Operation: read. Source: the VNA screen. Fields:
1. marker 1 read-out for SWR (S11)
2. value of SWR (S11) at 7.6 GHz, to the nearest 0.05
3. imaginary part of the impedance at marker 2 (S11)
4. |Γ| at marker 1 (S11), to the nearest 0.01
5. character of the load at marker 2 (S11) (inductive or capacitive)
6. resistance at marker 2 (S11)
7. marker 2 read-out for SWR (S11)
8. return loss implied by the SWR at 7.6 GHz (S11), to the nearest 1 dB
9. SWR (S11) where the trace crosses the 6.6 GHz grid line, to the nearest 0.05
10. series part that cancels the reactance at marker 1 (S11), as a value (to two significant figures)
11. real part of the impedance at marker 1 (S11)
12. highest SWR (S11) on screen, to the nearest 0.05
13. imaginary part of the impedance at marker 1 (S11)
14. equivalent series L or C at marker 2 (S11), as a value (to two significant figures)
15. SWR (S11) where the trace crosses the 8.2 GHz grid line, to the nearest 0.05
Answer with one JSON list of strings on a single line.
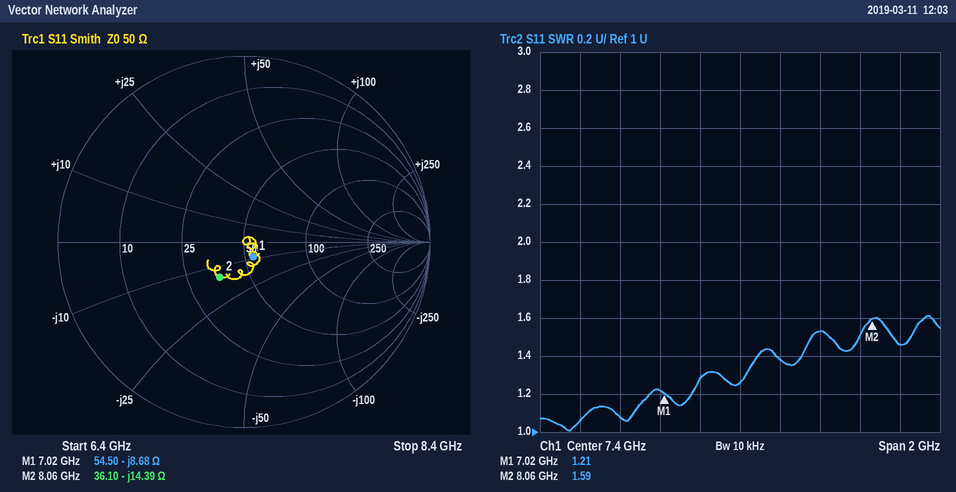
["1.21", "1.40", "-14.39 Ω", "0.09", "capacitive", "36.10 Ω", "1.59", "16 dB", "1.05", "200 pH", "54.50 Ω", "1.60", "-8.68 Ω", "1.4 pF", "1.45"]
